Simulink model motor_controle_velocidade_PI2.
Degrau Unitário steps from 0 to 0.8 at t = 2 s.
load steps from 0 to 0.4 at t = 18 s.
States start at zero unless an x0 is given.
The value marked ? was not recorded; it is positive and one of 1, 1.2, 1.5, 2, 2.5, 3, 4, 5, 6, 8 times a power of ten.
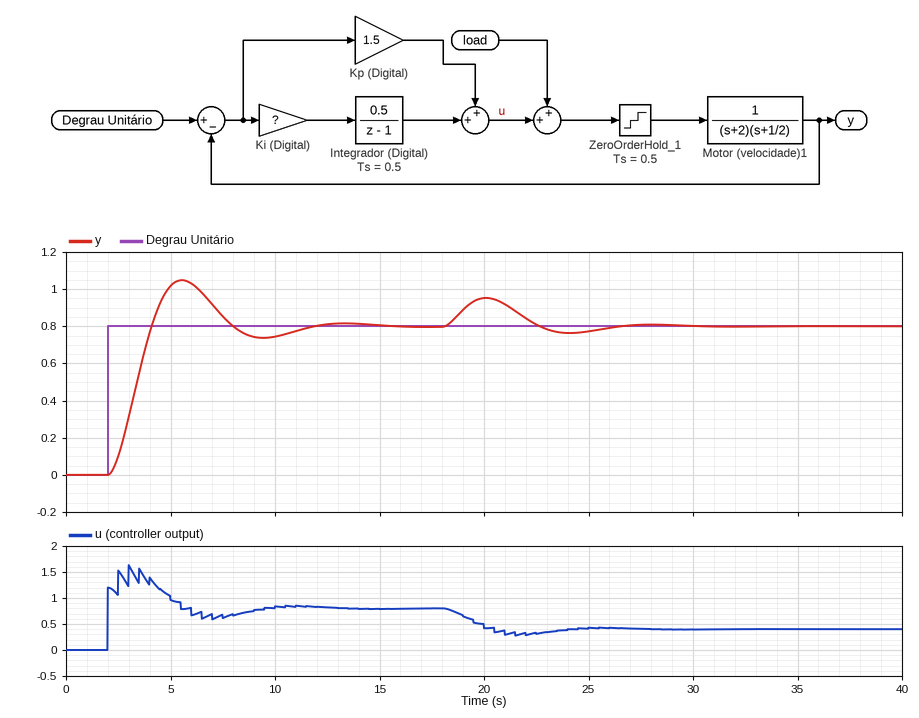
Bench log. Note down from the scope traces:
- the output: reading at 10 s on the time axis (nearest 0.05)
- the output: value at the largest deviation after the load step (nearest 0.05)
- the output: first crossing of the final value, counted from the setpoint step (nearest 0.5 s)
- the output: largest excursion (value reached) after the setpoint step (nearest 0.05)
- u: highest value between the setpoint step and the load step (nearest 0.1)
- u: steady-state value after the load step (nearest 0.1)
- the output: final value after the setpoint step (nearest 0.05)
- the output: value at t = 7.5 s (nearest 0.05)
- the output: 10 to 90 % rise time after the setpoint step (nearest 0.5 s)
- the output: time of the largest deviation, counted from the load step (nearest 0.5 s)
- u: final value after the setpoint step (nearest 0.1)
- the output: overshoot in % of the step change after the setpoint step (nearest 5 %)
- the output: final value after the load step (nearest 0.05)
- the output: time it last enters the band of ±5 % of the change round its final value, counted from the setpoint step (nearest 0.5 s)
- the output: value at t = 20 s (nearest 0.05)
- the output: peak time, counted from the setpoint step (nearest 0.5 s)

0.75
0.95
2.0 s
1.05
1.6
0.4
0.80
0.85
1.5 s
2.0 s
0.8
30 %
0.80
8.5 s
0.95
3.5 s
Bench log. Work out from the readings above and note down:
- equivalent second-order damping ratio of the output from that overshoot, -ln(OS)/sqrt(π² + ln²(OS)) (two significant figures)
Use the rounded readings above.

0.36
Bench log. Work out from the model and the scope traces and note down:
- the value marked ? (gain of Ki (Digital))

1.2
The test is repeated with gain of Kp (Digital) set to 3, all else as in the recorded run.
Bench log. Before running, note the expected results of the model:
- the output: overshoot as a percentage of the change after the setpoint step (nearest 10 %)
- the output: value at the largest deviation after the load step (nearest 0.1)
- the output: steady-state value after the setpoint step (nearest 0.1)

20 %
0.9
0.8
